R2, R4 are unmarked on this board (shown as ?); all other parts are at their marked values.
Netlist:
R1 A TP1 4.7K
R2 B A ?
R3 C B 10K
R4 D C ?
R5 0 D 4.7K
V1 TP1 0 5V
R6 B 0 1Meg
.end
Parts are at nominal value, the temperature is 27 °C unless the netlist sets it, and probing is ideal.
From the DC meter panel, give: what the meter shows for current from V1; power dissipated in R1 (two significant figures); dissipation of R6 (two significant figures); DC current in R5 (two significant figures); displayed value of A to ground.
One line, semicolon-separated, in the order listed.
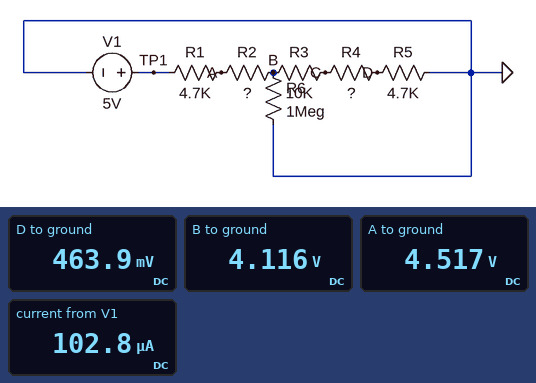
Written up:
102.8 µA; 50 µW; 17 µW; 99 µA; 4.517 V
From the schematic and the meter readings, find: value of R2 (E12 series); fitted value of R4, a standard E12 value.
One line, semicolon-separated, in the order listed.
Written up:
3.9 kΩ; 27 kΩ
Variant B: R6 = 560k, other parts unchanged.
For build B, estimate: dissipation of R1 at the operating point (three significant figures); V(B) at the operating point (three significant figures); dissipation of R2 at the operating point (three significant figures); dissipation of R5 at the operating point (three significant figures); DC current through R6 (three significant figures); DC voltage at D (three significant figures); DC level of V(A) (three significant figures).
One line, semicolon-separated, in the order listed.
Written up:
52.3 µW; 4.09 V; 43.4 µW; 45.3 µW; 7.31 µA; 461 mV; 4.50 V
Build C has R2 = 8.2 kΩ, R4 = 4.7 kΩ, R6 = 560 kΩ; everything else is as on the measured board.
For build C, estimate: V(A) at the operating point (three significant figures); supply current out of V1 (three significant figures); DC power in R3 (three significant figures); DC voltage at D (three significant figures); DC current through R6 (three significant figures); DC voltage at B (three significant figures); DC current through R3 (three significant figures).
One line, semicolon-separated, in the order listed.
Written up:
4.26 V; 158 µA; 233 µW; 718 mV; 5.29 µA; 2.96 V; 153 µA
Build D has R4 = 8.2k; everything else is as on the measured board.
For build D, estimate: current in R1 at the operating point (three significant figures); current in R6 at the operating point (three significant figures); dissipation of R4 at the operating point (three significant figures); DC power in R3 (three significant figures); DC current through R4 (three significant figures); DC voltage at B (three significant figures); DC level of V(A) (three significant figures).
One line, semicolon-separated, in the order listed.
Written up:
161 µA; 3.61 µA; 204 µW; 249 µW; 158 µA; 3.61 V; 4.24 V
